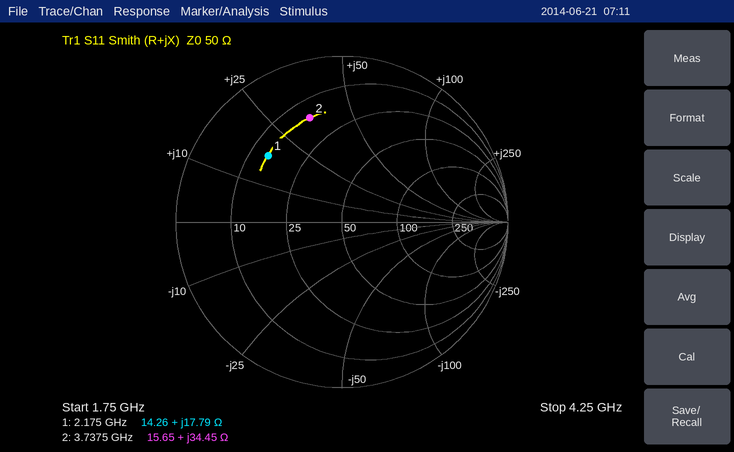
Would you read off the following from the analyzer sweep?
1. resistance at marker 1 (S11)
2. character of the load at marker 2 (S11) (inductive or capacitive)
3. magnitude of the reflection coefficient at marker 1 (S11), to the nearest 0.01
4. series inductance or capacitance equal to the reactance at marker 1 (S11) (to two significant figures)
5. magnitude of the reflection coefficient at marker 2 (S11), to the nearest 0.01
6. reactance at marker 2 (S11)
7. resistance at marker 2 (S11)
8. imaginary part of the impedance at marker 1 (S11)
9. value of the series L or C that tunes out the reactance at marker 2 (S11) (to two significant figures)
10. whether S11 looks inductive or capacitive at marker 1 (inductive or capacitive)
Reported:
14.26 Ω
inductive
0.60
1.3 nH
0.66
+34.45 Ω
15.65 Ω
+17.79 Ω
1.2 pF
inductive
